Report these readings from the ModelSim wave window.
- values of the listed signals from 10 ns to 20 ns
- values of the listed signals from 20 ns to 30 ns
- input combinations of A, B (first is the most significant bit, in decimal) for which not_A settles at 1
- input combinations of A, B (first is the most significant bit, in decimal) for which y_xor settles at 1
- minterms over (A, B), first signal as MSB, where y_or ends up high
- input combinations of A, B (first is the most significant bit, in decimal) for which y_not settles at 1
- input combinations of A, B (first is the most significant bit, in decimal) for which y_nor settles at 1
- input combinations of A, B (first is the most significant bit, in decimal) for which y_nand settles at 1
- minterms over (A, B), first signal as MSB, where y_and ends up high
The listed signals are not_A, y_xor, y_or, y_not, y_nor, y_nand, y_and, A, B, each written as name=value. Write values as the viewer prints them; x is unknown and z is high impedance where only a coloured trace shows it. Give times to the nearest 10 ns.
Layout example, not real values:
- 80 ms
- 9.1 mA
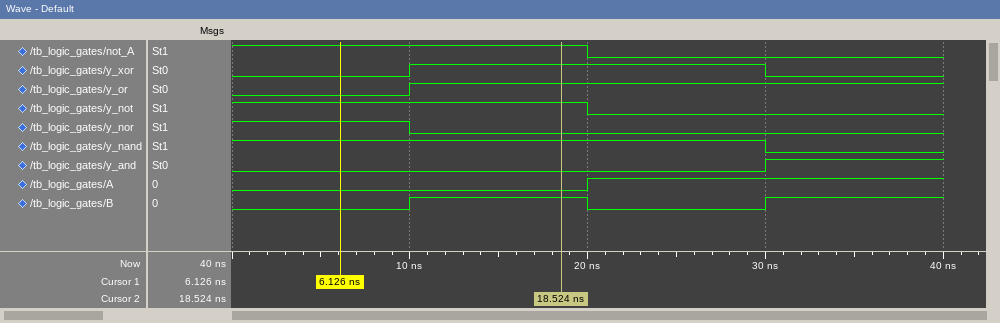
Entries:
- not_A=1, y_xor=1, y_or=1, y_not=1, y_nor=0, y_nand=1, y_and=0, A=0, B=1
- not_A=0, y_xor=1, y_or=1, y_not=0, y_nor=0, y_nand=1, y_and=0, A=1, B=0
- 0, 1
- 1, 2
- 1, 2, 3
- 0, 1
- 0
- 0, 1, 2
- 3
